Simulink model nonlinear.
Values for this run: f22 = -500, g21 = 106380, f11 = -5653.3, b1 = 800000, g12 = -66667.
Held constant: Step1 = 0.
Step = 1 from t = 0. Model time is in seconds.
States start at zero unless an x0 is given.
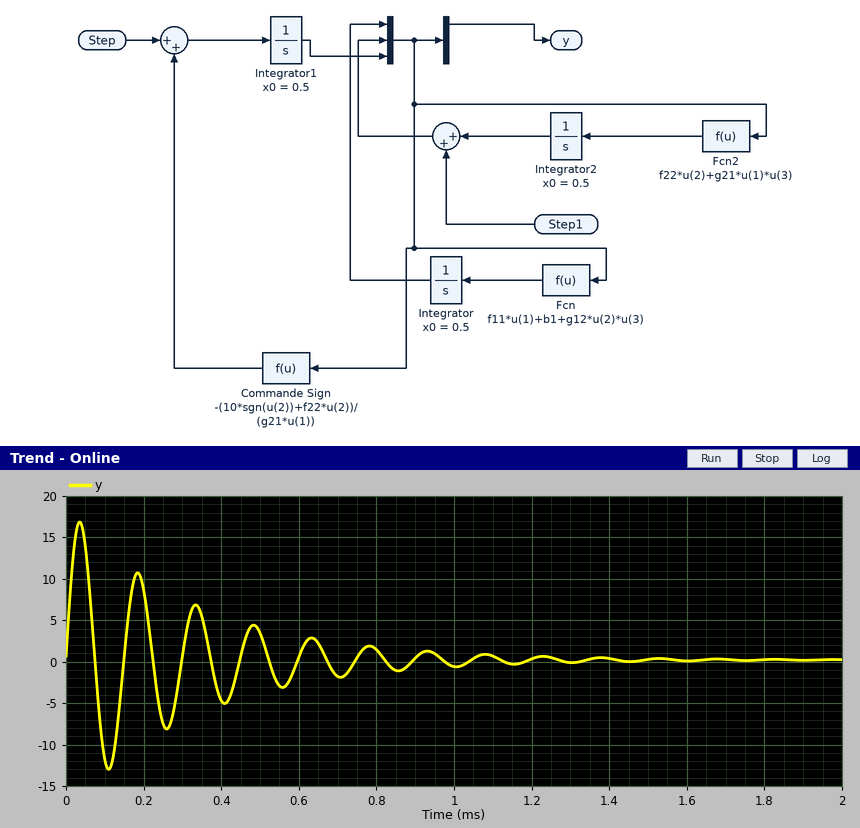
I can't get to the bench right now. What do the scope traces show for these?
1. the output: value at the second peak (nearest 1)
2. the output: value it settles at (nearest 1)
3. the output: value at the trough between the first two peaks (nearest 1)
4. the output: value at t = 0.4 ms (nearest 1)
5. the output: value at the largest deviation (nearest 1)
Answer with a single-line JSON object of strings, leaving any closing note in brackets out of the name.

{"the output: value at the second peak": "11", "the output: value it settles at": "0", "the output: value at the trough between the first two peaks": "-13", "the output: value at t = 0.4 ms": "-5", "the output: value at the largest deviation": "17"}
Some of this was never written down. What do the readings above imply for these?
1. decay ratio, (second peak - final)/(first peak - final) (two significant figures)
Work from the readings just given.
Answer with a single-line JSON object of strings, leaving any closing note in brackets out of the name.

{"decay ratio, (second peak - final)/(first peak - final)": "0.65"}
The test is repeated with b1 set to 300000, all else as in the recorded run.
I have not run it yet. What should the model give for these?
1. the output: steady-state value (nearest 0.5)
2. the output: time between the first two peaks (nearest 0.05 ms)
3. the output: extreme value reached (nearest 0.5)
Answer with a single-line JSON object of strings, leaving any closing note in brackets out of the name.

{"the output: steady-state value": "0.0", "the output: time between the first two peaks": "0.15 ms", "the output: extreme value reached": "6.0"}
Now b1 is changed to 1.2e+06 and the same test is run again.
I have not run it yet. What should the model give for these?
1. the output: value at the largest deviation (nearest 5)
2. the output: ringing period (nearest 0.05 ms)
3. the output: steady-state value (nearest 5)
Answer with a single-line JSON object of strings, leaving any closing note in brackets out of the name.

{"the output: value at the largest deviation": "25", "the output: ringing period": "0.15 ms", "the output: steady-state value": "0"}
